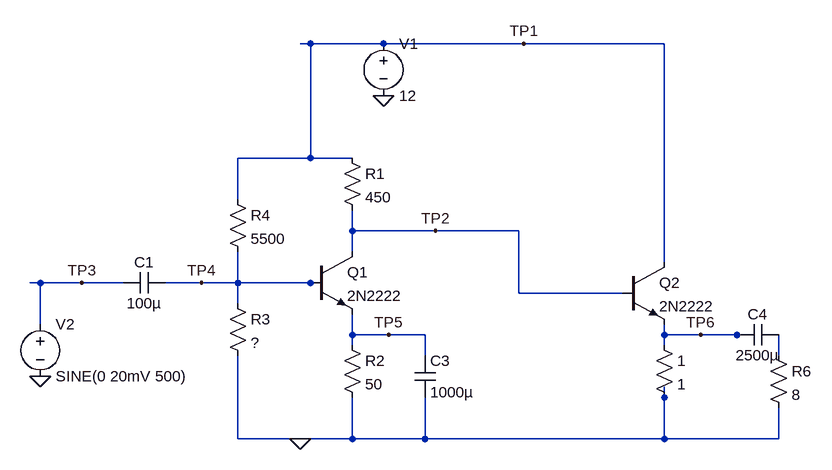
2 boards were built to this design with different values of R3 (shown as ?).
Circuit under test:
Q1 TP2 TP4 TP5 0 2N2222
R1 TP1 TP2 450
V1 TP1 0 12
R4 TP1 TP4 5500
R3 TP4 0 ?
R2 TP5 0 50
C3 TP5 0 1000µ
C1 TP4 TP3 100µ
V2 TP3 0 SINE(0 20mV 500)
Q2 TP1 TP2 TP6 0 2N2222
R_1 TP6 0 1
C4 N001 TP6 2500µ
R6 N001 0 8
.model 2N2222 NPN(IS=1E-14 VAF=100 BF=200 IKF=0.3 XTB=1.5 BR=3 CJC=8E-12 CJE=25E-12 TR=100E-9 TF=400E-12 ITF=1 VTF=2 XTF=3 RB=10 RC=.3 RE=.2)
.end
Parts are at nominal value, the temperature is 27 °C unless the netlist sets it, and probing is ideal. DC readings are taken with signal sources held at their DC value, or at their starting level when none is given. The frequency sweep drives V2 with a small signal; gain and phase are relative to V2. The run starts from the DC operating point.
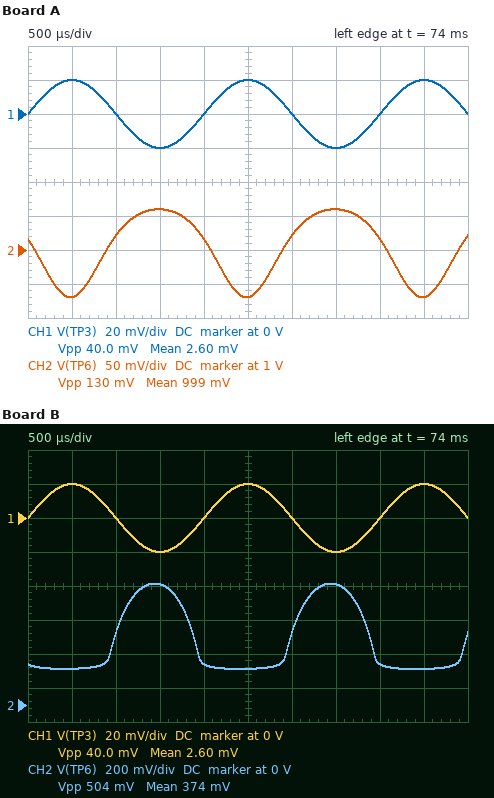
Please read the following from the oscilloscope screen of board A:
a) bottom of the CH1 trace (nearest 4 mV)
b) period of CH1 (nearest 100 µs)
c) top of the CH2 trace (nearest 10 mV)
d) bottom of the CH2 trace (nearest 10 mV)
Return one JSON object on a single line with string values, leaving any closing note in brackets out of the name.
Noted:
{"bottom of the CH1 trace": "-20 mV", "period of CH1": "2.0 ms", "top of the CH2 trace": "1.06 V", "bottom of the CH2 trace": "930 mV"}
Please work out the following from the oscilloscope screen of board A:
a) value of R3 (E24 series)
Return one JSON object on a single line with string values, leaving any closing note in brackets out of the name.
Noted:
{"value of R3": "430 Ω"}
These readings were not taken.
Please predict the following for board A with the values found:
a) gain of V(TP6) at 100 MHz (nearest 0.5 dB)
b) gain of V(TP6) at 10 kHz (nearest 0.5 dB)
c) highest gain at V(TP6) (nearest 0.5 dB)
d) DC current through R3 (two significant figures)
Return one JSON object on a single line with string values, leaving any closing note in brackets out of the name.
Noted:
{"gain of V(TP6) at 100 MHz": "-9.5 dB", "gain of V(TP6) at 10 kHz": "10.5 dB", "highest gain at V(TP6)": "10.5 dB", "DC current through R3": "2.0 mA"}
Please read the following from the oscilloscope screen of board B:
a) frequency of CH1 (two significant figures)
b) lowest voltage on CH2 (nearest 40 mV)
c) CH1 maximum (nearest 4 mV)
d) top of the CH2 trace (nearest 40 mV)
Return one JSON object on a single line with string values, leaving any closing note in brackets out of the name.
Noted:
{"frequency of CH1": "500 Hz", "lowest voltage on CH2": "200 mV", "CH1 maximum": "20 mV", "top of the CH2 trace": "720 mV"}
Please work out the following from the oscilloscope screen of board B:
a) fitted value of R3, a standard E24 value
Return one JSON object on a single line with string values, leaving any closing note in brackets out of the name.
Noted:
{"fitted value of R3, a standard E24 value": "1.2 kΩ"}
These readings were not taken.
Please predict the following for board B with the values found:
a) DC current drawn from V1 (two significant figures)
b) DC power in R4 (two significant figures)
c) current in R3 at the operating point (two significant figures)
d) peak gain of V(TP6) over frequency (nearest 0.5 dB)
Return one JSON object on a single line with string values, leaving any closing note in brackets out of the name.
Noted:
{"DC current drawn from V1": "320 mA", "DC power in R4": "19 mW", "current in R3 at the operating point": "1.5 mA", "peak gain of V(TP6) over frequency": "13.5 dB"}
